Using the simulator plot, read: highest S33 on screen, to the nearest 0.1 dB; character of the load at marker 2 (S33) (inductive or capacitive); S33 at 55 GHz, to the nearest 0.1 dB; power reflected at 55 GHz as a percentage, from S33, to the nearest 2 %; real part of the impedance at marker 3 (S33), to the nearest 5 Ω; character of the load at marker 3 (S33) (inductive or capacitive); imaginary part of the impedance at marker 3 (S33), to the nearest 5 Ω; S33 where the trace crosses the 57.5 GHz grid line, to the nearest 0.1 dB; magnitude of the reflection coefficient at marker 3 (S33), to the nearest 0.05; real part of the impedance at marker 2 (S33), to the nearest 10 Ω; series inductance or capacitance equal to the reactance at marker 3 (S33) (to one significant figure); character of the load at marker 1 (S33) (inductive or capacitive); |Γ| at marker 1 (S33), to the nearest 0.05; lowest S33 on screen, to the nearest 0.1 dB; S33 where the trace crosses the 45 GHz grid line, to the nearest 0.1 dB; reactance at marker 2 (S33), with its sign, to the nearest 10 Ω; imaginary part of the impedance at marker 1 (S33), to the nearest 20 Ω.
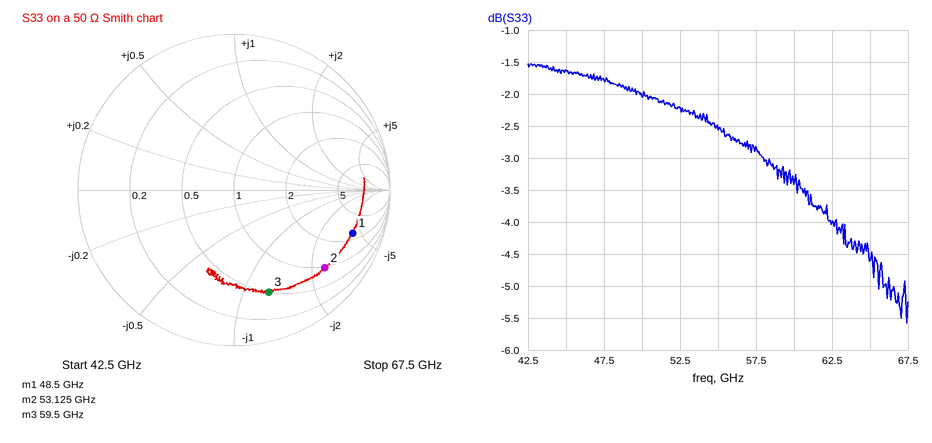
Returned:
-1.5 dB
capacitive
-2.5 dB
56 %
25 Ω
capacitive
-65 Ω
-2.8 dB
0.70
50 Ω
40 fF
capacitive
0.80
-5.6 dB
-1.6 dB
-120 Ω
-200 Ω
